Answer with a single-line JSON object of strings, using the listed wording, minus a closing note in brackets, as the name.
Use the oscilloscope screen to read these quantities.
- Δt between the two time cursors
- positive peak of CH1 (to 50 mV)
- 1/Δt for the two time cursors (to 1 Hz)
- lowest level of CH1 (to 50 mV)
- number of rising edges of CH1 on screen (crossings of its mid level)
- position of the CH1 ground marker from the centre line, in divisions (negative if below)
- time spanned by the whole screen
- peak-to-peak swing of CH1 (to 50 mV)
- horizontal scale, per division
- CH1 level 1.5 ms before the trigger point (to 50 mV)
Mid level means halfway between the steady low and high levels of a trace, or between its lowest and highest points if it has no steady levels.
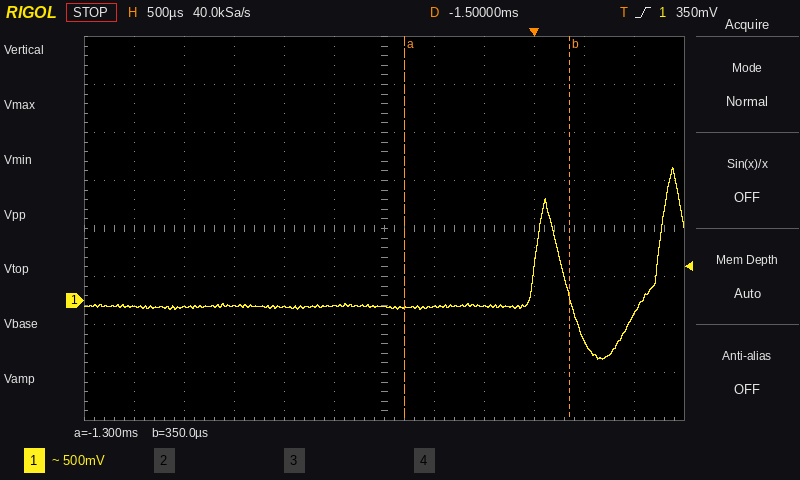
{"Δt between the two time cursors": "1.65 ms", "positive peak of CH1": "1.40 V", "1/Δt for the two time cursors": "606 Hz", "lowest level of CH1": "-600 mV", "number of rising edges of CH1 on screen": "2", "position of the CH1 ground marker from the centre line, in divisions": "-1.5 div", "time spanned by the whole screen": "6 ms", "peak-to-peak swing of CH1": "2.00 V", "horizontal scale, per division": "500 µs", "CH1 level 1.5 ms before the trigger point": "-50 mV"}
